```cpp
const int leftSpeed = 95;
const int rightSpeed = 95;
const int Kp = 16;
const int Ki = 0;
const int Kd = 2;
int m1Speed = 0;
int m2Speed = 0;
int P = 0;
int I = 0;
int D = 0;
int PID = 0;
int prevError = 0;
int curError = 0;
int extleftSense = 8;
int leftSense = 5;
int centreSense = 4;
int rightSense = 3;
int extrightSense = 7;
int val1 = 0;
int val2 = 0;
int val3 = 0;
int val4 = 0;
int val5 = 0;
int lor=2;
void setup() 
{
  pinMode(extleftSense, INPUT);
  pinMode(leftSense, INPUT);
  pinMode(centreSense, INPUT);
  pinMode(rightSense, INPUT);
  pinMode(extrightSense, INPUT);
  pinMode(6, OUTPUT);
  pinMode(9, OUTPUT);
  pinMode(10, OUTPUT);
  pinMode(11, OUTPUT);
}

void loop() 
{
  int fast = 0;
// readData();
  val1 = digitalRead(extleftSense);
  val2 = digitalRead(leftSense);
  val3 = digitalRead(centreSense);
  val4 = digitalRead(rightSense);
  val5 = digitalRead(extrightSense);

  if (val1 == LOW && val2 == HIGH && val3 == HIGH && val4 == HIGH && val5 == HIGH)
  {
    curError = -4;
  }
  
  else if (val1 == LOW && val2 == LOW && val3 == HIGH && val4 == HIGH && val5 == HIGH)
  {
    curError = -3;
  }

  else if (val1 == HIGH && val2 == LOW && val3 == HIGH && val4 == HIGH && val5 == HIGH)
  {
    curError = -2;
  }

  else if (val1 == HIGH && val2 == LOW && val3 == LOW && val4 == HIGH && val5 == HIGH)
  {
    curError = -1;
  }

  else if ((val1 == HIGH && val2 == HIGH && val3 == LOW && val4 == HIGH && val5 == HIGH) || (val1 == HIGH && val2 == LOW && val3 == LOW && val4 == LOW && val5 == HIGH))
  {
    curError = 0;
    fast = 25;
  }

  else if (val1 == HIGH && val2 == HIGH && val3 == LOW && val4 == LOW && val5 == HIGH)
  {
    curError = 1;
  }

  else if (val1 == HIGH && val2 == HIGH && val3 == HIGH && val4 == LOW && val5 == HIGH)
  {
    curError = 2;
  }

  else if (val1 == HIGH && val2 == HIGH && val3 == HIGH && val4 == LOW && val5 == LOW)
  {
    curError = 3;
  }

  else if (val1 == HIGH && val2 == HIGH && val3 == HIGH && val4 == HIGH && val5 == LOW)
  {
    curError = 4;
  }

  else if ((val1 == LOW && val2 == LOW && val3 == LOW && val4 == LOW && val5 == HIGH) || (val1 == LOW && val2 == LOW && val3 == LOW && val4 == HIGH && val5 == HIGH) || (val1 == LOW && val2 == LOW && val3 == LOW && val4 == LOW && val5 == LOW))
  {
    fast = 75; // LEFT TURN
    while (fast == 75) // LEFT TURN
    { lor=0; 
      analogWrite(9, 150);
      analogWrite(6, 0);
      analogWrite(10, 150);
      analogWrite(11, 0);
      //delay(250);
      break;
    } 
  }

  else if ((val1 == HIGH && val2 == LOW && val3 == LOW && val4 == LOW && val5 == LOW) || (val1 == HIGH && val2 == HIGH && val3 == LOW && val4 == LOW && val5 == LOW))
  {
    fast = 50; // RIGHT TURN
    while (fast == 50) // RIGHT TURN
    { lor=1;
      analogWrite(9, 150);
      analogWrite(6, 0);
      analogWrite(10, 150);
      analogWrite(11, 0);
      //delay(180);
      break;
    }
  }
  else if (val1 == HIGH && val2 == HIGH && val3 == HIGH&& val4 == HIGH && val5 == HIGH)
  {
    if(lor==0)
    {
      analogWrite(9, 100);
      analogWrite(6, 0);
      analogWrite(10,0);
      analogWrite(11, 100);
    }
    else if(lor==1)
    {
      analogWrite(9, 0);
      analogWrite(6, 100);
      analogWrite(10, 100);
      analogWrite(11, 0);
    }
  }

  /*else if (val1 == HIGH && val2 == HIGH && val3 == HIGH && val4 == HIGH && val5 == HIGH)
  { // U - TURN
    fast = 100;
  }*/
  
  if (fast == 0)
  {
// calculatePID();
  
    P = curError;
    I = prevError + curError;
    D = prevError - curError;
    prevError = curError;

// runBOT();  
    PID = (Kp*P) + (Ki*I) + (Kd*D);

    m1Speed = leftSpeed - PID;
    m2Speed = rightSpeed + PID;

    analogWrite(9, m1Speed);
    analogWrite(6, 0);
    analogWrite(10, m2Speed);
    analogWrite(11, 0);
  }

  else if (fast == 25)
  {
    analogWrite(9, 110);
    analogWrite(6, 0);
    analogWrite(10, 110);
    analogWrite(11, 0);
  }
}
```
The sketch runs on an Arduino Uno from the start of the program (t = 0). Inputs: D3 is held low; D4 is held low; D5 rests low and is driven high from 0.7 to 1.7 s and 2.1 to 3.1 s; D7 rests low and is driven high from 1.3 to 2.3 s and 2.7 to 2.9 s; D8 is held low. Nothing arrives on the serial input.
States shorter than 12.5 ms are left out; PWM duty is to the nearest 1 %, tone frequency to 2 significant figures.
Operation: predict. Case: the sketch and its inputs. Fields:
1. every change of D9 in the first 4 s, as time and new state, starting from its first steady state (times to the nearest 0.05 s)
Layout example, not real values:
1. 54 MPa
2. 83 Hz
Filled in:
1. 0 s PWM 59 %; 0.7 s PWM 37 %; 1.7 s PWM 59 %; 2.1 s PWM 37 %; 3.1 s PWM 59 %
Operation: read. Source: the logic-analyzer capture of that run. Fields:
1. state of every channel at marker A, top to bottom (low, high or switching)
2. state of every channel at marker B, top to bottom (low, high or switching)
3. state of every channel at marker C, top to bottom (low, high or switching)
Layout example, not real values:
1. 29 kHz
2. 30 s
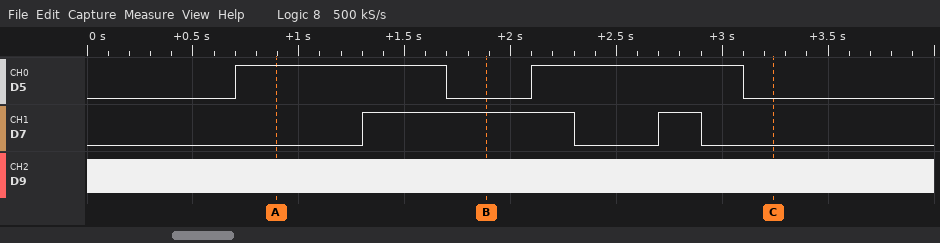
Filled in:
1. D5 high, D7 low, D9 switching
2. D5 low, D7 high, D9 switching
3. D5 low, D7 low, D9 switching
